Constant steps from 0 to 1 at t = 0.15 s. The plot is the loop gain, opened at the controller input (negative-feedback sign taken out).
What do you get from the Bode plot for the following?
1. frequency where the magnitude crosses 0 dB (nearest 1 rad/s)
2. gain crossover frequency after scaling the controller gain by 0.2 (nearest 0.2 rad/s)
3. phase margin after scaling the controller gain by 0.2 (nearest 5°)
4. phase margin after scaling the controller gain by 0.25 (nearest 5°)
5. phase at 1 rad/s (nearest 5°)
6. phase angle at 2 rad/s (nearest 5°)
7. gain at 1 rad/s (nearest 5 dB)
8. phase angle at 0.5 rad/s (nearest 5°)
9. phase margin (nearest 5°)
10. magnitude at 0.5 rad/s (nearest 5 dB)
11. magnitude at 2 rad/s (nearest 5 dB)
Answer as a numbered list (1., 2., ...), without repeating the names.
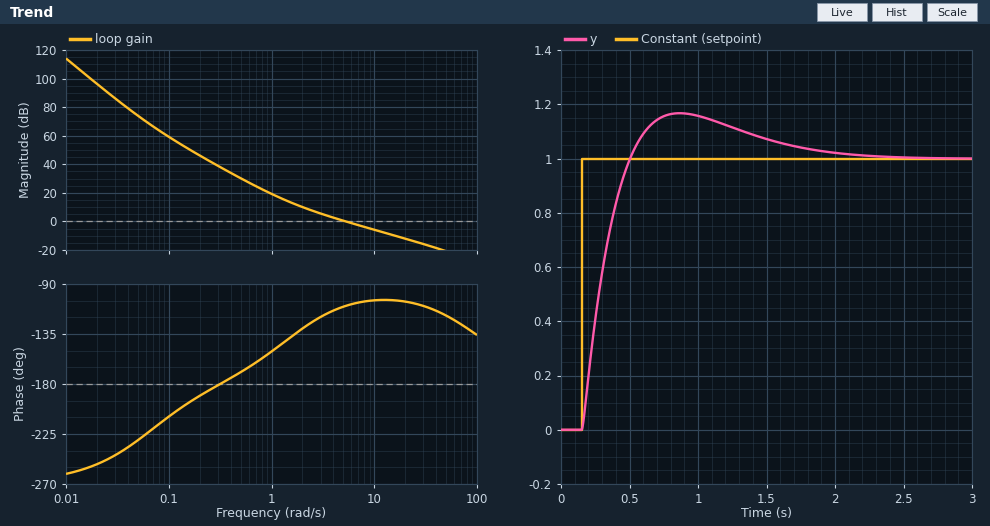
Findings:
1. 5 rad/s
2. 1.4 rad/s
3. 40°
4. 45°
5. -150°
6. -130°
7. 20 dB
8. -170°
9. 70°
10. 30 dB
11. 10 dB
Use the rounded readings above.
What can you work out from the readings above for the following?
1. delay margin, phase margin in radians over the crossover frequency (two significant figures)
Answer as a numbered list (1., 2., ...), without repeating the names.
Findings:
1. 0.24 s
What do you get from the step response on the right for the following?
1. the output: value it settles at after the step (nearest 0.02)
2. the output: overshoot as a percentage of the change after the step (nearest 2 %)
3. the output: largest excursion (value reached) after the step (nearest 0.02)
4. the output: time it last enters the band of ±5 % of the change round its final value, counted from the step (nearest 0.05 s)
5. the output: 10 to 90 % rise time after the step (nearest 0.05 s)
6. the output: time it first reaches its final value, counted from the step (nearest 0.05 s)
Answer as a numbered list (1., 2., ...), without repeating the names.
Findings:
1. 1.00
2. 16 %
3. 1.16
4. 1.50 s
5. 0.25 s
6. 0.35 s
